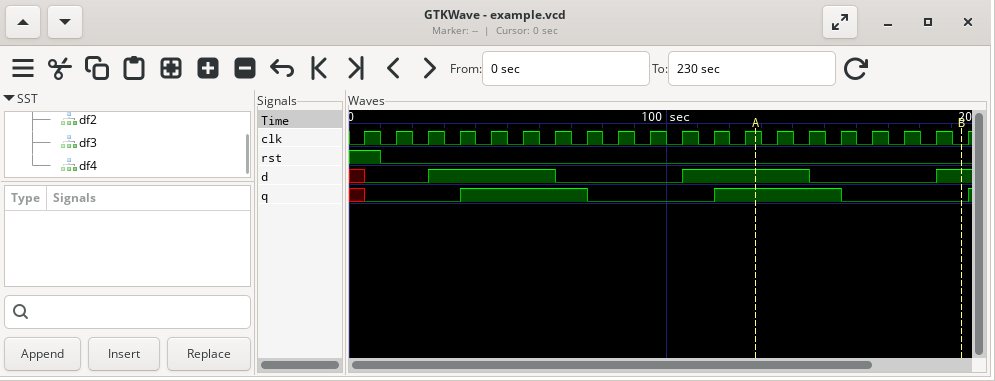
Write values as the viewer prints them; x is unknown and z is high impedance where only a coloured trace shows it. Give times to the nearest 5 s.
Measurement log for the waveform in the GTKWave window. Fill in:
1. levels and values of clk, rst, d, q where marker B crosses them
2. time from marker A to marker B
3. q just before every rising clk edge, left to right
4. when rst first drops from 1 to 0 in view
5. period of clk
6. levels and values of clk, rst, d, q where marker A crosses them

clk=0, rst=0, d=1, q=0
65 s
x 0 0 0 1 1 1 1 0 0 0 0 1 1 1 1 0 0 0 0
10 s
10 s
clk=1, rst=0, d=1, q=1
